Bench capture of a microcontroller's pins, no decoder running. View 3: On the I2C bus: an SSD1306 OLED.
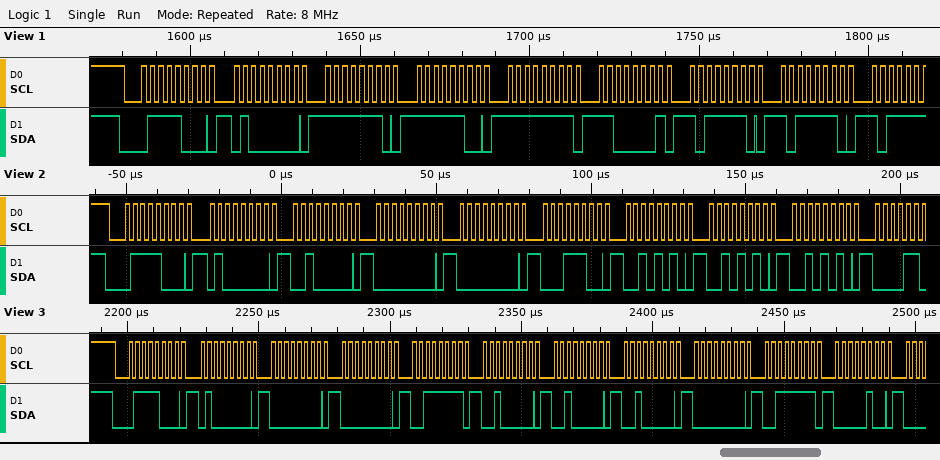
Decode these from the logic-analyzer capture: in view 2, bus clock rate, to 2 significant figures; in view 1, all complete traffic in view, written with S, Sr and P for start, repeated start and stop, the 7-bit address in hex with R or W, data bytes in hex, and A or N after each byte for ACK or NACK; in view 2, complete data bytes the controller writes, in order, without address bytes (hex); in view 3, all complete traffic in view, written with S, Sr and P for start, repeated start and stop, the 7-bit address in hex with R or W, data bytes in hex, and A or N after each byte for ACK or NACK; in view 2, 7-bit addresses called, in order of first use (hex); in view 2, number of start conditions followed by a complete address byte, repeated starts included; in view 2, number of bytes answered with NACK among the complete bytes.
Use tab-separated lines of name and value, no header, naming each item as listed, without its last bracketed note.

in view 2, bus clock rate, to 2 significant figures	400 kHz
in view 1, all complete traffic in view, written with S, Sr and P for start, repeated start and stop, the 7-bit address in hex with R or W, data bytes in hex, and A or N after each byte for ACK or NACK	S 3CW A 40 A FE A FC A FF A C1 A BE A BE A
in view 2, complete data bytes the controller writes, in order, without address bytes	40 20 00 00 1C 2A 2A 2A
in view 3, all complete traffic in view, written with S, Sr and P for start, repeated start and stop, the 7-bit address in hex with R or W, data bytes in hex, and A or N after each byte for ACK or NACK	S 3CW A 40 A 00 A 00 A 3F A 20 A 20 A 20 A 00 A 3F A 04 A
in view 2, 7-bit addresses called, in order of first use	0x3C
in view 2, number of start conditions followed by a complete address byte, repeated starts included	1
in view 2, number of bytes answered with NACK among the complete bytes	0
